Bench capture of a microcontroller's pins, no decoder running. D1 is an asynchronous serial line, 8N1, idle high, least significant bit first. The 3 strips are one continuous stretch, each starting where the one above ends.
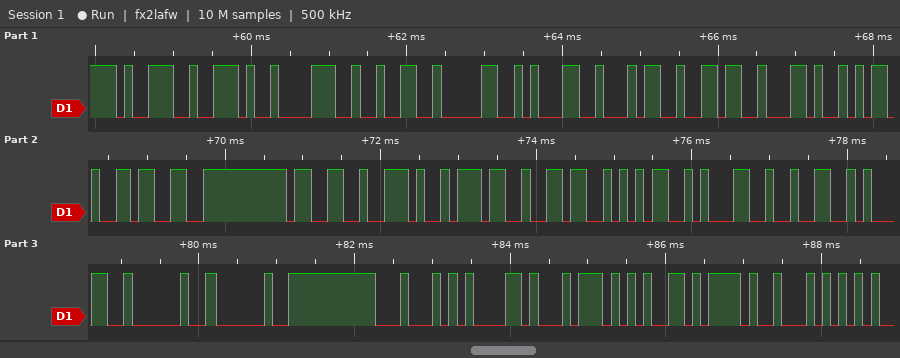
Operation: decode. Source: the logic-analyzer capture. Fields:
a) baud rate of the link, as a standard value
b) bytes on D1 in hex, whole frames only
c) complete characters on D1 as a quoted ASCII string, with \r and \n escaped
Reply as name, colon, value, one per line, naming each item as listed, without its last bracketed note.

baud rate of the link, as a standard value: 9600 baud
bytes on D1 in hex, whole frames only: 0x39 0x2E 0x38 0x32 0x30 0x31 0x34 0x36 0x2C 0x2D 0x33 0x33 0x2E 0x37 0x36 0x35 0x31 0x32 0x31 0x20 0x20 0x44 0x61 0x74 0x65 0x2F 0x54
complete characters on D1 as a quoted ASCII string, with \r and \n escaped: "9.820146,-33.765121  Date/T"
